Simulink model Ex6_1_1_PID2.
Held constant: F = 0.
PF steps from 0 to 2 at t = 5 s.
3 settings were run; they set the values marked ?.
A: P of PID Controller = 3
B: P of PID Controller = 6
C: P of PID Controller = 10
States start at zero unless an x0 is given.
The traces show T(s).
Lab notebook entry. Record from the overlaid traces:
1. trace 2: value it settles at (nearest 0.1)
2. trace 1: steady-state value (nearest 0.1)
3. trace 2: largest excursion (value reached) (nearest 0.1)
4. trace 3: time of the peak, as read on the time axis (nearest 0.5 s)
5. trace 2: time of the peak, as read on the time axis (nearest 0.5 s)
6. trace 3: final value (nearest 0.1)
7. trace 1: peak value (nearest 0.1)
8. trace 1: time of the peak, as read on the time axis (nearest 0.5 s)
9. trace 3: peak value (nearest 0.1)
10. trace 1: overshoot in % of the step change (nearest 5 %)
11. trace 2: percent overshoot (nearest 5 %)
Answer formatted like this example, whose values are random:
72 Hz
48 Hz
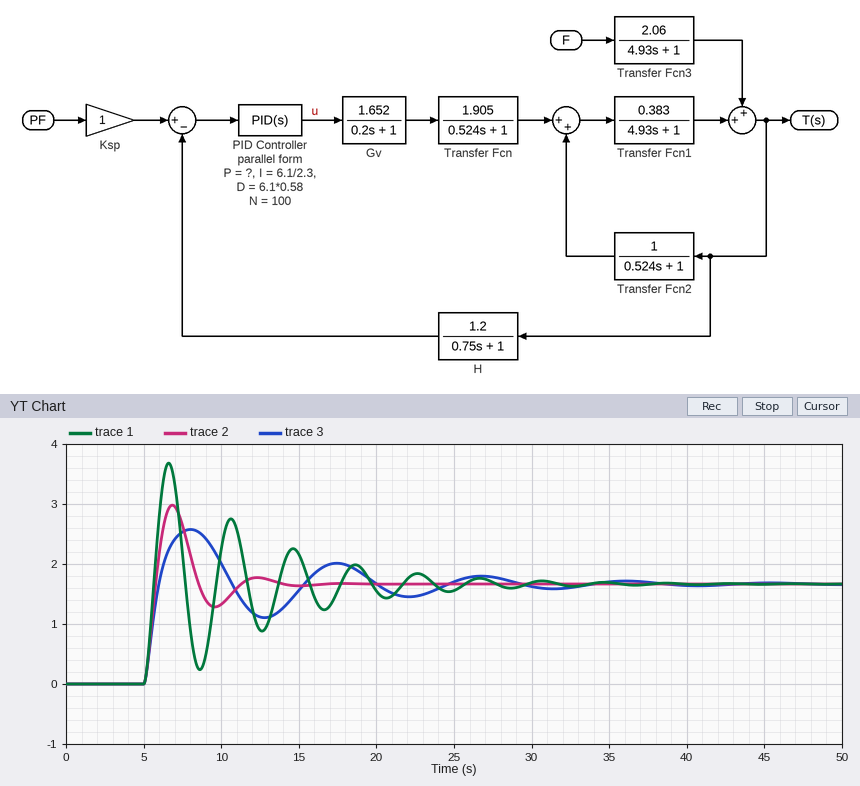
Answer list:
1.7
1.7
3.0
8.0 s
7.0 s
1.7
3.7
6.5 s
2.6
120 %
80 %
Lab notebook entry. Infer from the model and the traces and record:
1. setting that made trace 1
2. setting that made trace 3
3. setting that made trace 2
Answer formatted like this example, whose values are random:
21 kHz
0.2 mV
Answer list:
C
A
B
